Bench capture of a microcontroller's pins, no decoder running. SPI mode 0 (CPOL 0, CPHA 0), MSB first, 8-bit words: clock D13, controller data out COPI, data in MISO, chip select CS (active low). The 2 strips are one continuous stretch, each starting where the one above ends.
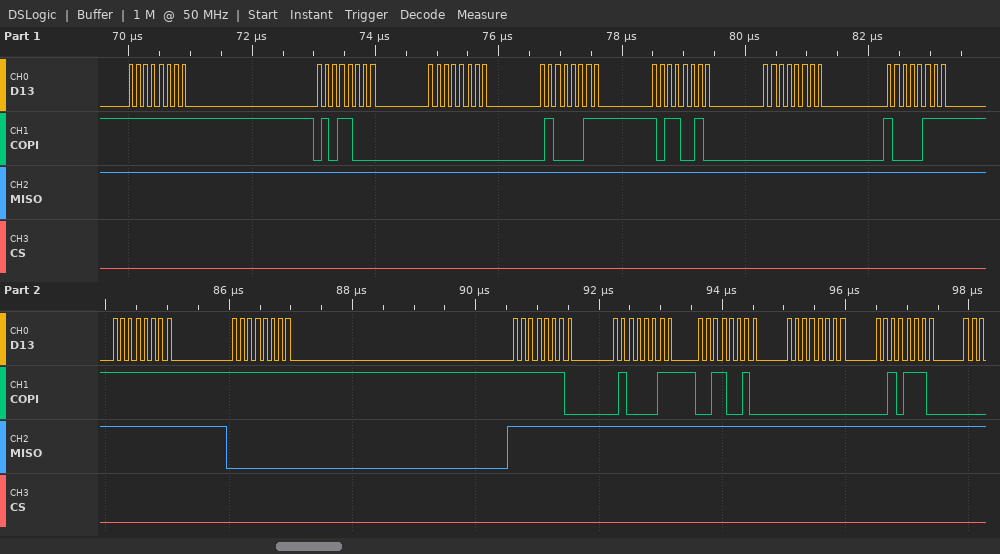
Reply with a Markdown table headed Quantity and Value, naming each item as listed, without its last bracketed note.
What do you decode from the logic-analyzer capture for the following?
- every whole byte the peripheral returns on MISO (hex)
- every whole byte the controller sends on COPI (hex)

| Quantity | Value |
|---|---|
| every whole byte the peripheral returns on MISO | FF FF FF FF FF FF FF FF 00 FF FF FF FF FF |
| every whole byte the controller sends on COPI | FF 58 00 43 B2 00 87 FF FF FE 43 32 00 2E |
